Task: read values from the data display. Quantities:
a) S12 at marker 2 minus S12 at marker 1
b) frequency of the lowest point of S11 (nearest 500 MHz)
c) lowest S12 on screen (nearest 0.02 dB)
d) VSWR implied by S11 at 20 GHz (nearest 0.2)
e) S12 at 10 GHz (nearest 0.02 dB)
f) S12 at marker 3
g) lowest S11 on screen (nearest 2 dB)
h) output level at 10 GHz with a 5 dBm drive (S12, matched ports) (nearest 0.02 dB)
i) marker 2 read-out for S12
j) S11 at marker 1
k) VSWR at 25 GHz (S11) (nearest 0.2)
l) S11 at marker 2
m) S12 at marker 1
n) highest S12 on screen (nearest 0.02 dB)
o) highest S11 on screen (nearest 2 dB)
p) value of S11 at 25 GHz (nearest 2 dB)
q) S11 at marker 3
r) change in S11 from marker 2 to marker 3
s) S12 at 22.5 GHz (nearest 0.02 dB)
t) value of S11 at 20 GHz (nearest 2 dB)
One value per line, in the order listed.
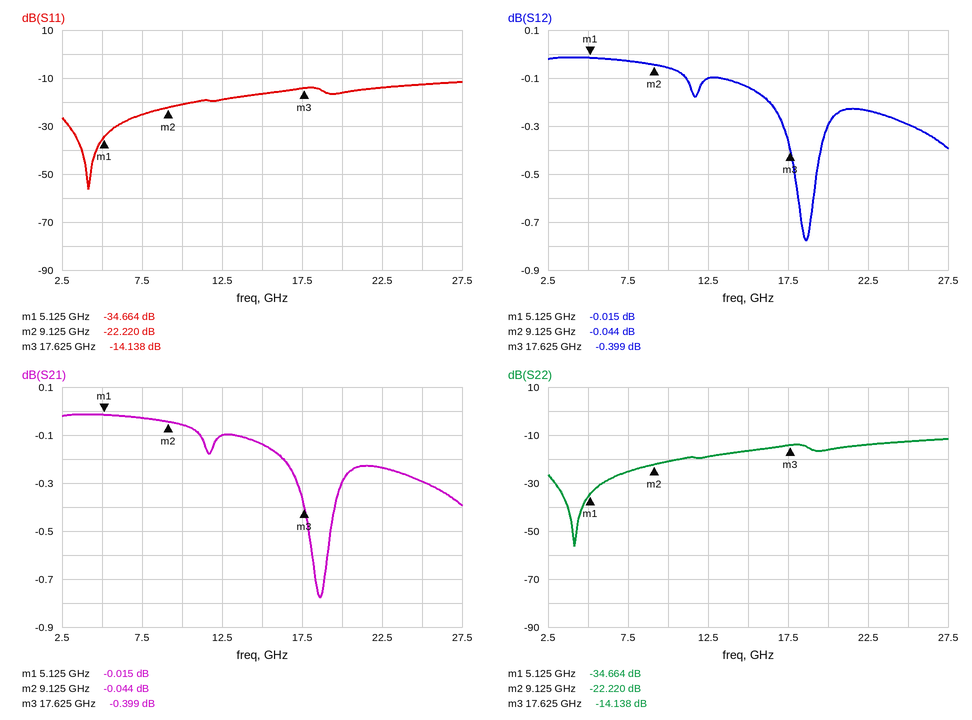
-0.029 dB
4.0 GHz
-0.78 dB
1.4
-0.06 dB
-0.399 dB
-56 dB
4.94 dBm
-0.044 dB
-34.664 dB
1.6
-22.220 dB
-0.015 dB
-0.02 dB
-12 dB
-12 dB
-14.138 dB
8.082 dB
-0.24 dB
-16 dB
